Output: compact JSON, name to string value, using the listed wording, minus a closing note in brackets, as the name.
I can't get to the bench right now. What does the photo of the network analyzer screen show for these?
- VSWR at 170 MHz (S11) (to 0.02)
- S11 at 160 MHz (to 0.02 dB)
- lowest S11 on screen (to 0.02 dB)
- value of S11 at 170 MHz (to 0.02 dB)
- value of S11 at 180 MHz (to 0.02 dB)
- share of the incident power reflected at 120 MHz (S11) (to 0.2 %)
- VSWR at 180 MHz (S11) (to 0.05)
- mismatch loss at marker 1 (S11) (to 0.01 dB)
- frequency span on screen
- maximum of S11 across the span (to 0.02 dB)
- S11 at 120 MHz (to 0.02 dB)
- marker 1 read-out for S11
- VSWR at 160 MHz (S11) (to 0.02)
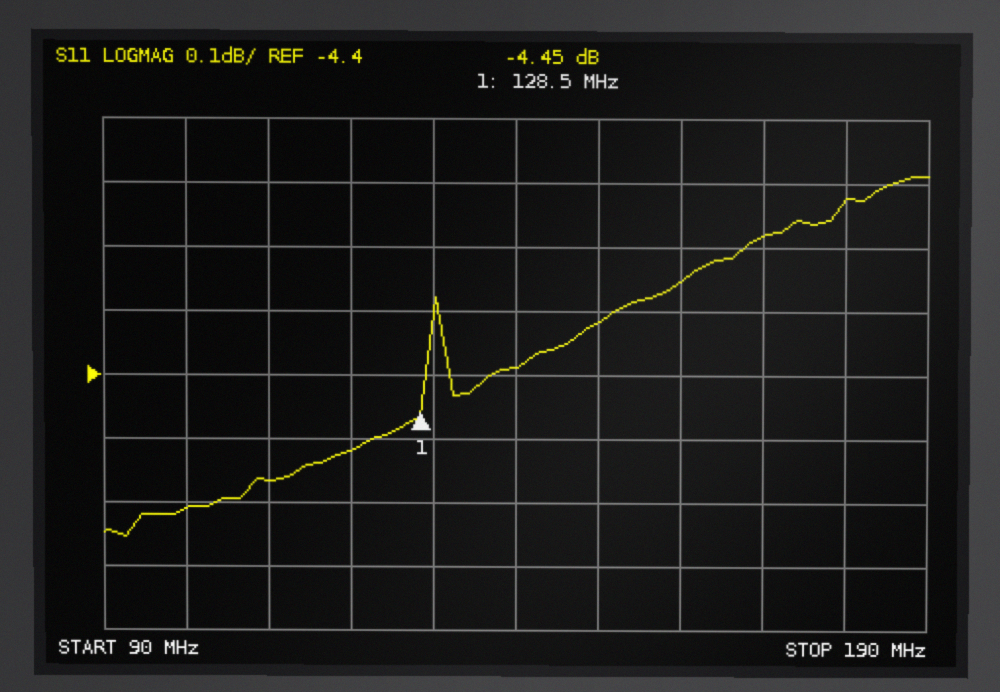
{"VSWR at 170 MHz (S11)": "4.24", "S11 at 160 MHz": "-4.26 dB", "lowest S11 on screen": "-4.66 dB", "value of S11 at 170 MHz": "-4.18 dB", "value of S11 at 180 MHz": "-4.12 dB", "share of the incident power reflected at 120 MHz (S11)": "35.4 %", "VSWR at 180 MHz (S11)": "4.30", "mismatch loss at marker 1 (S11)": "1.93 dB", "frequency span on screen": "100 MHz", "maximum of S11 across the span": "-4.08 dB", "S11 at 120 MHz": "-4.52 dB", "marker 1 read-out for S11": "-4.45 dB", "VSWR at 160 MHz (S11)": "4.16"}
